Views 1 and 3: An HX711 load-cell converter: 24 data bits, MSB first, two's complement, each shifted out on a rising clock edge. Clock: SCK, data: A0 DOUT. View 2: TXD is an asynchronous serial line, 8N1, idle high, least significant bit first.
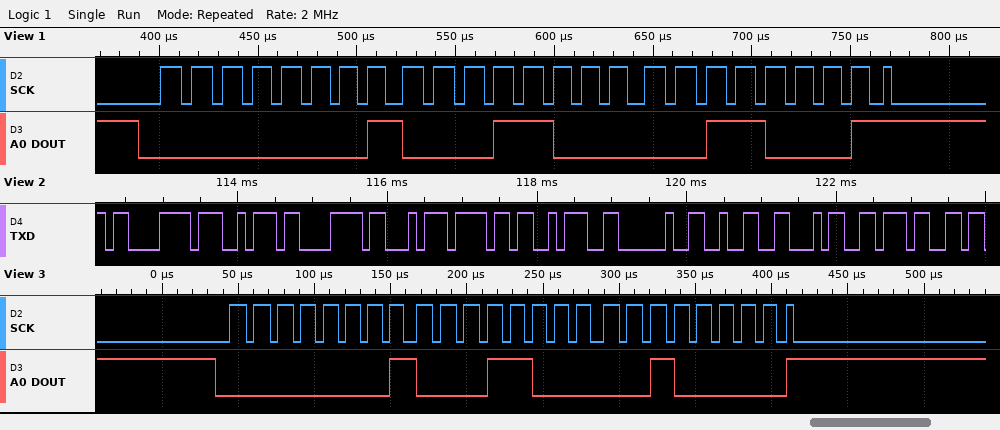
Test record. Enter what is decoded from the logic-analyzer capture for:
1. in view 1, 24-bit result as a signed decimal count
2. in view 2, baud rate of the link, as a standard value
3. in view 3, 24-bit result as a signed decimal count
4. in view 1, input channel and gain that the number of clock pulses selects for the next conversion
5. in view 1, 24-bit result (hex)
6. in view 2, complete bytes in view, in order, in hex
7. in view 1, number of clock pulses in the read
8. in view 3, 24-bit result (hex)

71729
9600 baud
71712
channel A, gain 128
0x011831
C3 A7 C3 A3 6F 3A 20 32 34 37
25
0x011820
